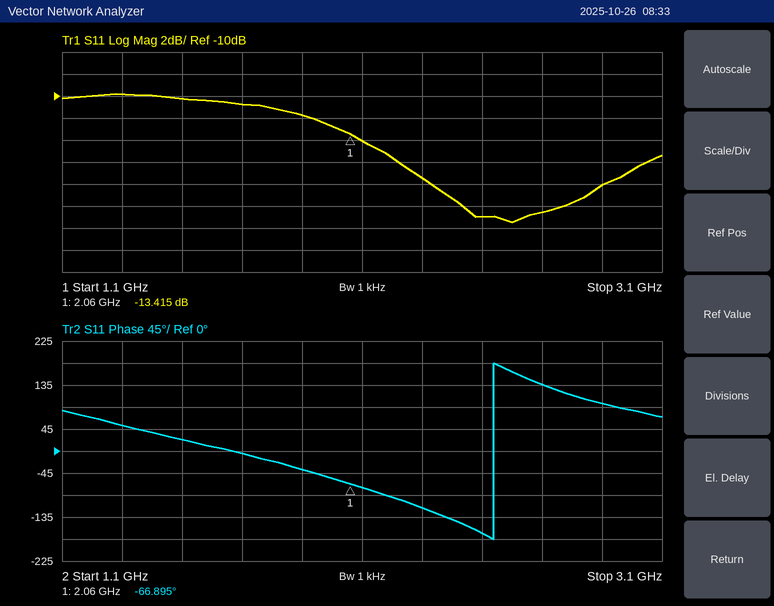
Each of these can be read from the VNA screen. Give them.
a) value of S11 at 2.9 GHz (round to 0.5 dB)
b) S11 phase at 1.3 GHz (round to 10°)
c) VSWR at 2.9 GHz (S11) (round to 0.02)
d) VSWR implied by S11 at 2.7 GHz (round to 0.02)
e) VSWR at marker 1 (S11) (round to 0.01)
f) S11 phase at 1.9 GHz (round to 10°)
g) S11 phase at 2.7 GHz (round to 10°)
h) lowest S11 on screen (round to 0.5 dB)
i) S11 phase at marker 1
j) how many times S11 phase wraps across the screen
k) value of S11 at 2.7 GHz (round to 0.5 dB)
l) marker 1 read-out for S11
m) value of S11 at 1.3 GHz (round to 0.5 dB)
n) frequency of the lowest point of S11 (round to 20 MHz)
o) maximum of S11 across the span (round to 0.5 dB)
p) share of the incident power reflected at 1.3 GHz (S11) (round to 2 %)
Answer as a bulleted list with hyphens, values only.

- -18.0 dB
- 50°
- 1.28
- 1.20
- 1.54
- -40°
- 140°
- -21.5 dB
- -66.895°
- 1
- -20.5 dB
- -13.415 dB
- -10.0 dB
- 2.60 GHz
- -10.0 dB
- 10 %
